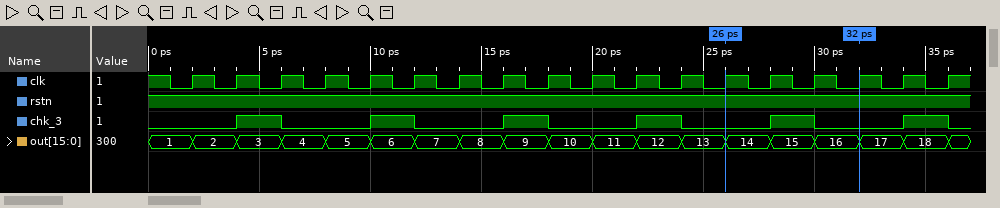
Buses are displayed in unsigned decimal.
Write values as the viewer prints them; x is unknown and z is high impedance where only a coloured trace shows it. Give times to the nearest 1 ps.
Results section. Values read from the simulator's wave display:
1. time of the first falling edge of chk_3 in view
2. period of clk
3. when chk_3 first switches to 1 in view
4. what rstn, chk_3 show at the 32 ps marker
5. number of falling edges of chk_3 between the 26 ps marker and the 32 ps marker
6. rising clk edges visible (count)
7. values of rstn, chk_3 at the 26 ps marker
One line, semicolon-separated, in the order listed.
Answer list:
6 ps; 2 ps; 4 ps; rstn=1, chk_3=0; 1; 18; rstn=1, chk_3=0
